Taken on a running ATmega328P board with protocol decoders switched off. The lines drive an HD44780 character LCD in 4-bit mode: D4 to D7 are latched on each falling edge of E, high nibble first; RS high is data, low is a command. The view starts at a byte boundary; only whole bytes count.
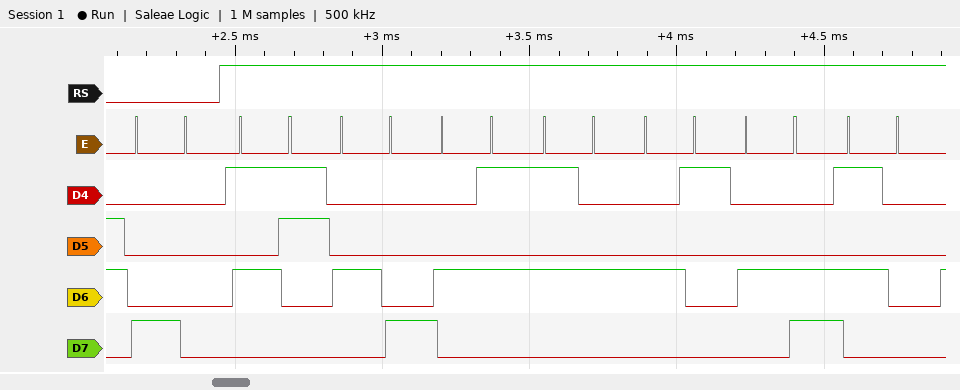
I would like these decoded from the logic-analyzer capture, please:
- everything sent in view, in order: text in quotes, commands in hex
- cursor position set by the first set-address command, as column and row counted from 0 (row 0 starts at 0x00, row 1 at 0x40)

0x80 "SHETALP"
column 0, row 0
